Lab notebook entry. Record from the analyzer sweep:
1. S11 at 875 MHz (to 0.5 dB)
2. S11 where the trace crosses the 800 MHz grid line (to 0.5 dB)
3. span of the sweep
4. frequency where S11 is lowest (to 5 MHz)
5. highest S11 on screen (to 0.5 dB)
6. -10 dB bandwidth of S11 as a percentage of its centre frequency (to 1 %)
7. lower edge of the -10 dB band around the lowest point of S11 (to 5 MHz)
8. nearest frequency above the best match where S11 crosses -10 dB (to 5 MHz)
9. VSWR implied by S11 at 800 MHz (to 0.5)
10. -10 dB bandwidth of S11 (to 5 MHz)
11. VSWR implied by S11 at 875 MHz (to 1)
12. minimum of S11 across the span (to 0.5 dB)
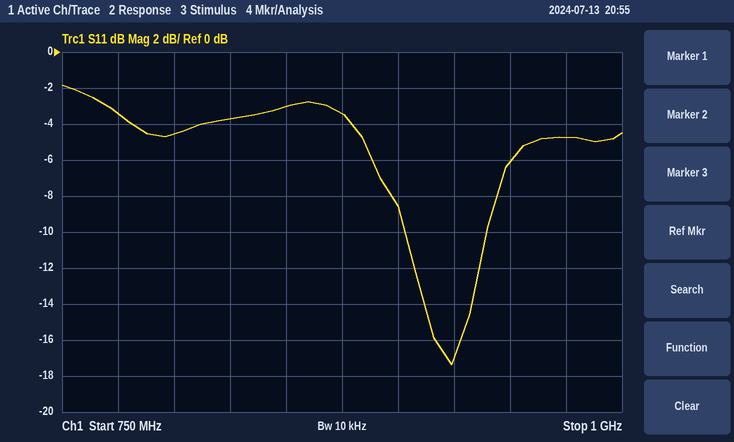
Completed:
-3.5 dB
-4.5 dB
250 MHz
925 MHz
-2.0 dB
4 %
905 MHz
940 MHz
4.0
35 MHz
5
-17.5 dB
